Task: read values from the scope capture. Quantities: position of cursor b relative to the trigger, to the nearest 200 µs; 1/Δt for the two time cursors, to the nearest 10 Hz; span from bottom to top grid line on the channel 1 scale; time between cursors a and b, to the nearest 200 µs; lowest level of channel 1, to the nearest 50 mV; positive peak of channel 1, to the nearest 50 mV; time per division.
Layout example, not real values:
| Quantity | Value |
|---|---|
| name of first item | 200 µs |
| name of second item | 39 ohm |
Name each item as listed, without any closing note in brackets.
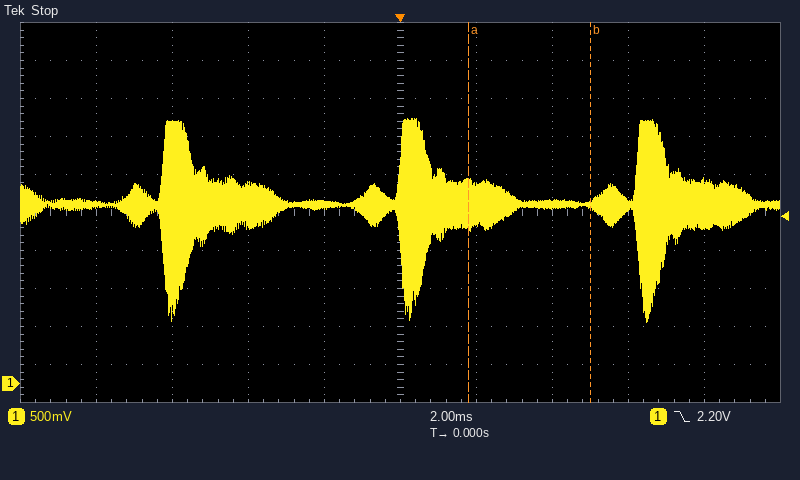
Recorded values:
| Quantity | Value |
|---|---|
| position of cursor b relative to the trigger, to the nearest 200 µs | +5.0 ms |
| 1/Δt for the two time cursors, to the nearest 10 Hz | 310 Hz |
| span from bottom to top grid line on the channel 1 scale | 5 V |
| time between cursors a and b, to the nearest 200 µs | 3.2 ms |
| lowest level of channel 1, to the nearest 50 mV | 800 mV |
| positive peak of channel 1, to the nearest 50 mV | 3.50 V |
| time per division | 2 ms |
